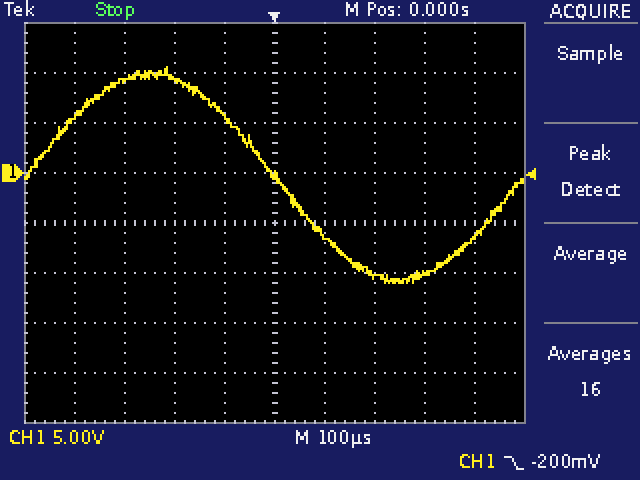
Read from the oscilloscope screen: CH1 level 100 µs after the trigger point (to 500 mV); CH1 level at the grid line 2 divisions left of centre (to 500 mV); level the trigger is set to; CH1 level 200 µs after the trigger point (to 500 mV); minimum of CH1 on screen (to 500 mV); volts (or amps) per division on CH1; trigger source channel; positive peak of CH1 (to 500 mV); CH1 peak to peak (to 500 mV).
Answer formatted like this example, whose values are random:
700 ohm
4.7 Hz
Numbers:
-6.0 V
9.5 V
-200 mV
-10.0 V
-11.0 V
5 V
CH1
10.5 V
21.5 V
